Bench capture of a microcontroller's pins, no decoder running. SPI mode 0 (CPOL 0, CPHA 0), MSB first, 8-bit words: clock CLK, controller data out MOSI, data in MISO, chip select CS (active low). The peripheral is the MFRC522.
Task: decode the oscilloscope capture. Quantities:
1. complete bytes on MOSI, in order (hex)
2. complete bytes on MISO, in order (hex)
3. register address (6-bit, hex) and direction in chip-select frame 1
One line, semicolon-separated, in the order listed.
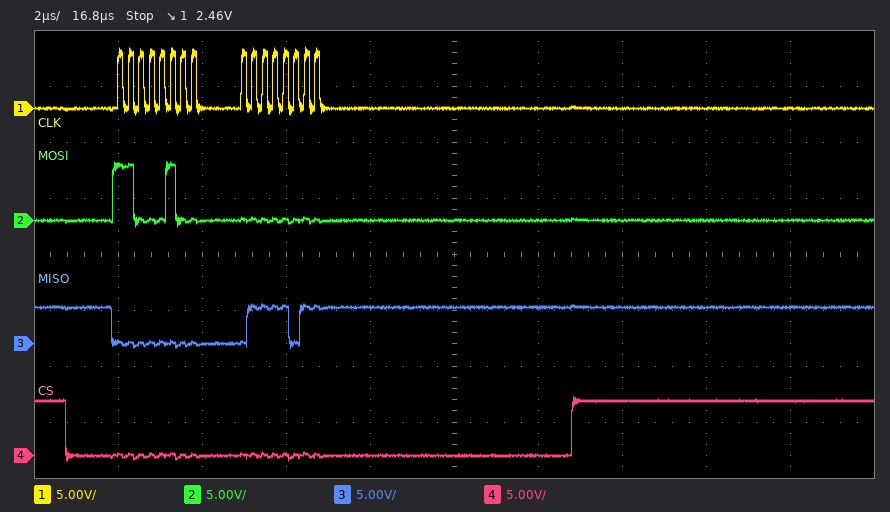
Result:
C4 00; 00 7B; 0x22 read
